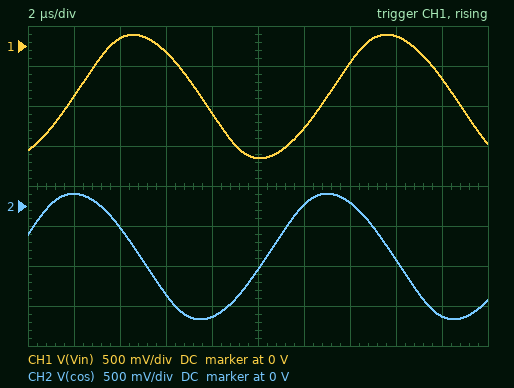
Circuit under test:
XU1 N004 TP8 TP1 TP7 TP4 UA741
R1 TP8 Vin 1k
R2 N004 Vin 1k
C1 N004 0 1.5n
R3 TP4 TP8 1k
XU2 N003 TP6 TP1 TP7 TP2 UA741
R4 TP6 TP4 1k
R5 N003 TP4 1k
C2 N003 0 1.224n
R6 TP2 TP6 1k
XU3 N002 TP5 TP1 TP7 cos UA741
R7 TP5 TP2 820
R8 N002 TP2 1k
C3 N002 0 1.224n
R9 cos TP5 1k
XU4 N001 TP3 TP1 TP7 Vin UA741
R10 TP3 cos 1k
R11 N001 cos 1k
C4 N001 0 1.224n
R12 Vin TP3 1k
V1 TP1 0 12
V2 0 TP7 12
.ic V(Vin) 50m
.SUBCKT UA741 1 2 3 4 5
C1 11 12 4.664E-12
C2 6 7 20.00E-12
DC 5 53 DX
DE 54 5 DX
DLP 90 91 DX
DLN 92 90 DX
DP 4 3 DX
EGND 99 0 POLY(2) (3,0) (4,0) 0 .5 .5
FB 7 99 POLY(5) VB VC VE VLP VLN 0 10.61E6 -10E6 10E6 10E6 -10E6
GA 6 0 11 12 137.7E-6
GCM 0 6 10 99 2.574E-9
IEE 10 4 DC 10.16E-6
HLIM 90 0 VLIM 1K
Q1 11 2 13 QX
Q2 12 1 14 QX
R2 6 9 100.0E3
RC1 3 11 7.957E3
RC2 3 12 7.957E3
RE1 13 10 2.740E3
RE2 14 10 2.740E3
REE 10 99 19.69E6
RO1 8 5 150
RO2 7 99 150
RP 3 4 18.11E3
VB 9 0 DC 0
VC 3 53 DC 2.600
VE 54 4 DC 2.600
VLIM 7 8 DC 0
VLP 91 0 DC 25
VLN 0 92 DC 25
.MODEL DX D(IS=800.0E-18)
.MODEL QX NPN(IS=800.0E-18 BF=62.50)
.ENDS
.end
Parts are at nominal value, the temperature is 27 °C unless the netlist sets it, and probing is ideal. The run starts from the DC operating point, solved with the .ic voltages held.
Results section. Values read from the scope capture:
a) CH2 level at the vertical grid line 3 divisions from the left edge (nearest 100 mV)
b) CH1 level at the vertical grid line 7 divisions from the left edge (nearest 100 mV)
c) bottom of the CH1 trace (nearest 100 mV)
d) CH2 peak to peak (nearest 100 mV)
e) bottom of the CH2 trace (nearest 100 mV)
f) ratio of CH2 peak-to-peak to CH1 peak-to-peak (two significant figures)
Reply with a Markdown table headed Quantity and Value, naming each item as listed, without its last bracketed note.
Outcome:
| Quantity | Value |
|---|---|
| CH2 level at the vertical grid line 3 divisions from the left edge | -1.1 V |
| CH1 level at the vertical grid line 7 divisions from the left edge | -200 mV |
| bottom of the CH1 trace | -1.4 V |
| CH2 peak to peak | 1.6 V |
| bottom of the CH2 trace | -1.4 V |
| ratio of CH2 peak-to-peak to CH1 peak-to-peak | 1.0 |
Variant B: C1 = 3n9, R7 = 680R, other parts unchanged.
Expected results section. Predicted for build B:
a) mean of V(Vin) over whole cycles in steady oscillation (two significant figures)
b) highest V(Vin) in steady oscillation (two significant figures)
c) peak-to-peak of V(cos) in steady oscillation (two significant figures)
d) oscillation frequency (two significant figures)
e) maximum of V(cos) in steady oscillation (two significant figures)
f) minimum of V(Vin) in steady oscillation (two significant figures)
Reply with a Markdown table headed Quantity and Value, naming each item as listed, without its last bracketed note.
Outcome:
| Quantity | Value |
|---|---|
| mean of V(Vin) over whole cycles in steady oscillation | -390 mV |
| highest V(Vin) in steady oscillation | 720 mV |
| peak-to-peak of V(cos) in steady oscillation | 2.3 V |
| oscillation frequency | 70 kHz |
| maximum of V(cos) in steady oscillation | 760 mV |
| minimum of V(Vin) in steady oscillation | -1.5 V |
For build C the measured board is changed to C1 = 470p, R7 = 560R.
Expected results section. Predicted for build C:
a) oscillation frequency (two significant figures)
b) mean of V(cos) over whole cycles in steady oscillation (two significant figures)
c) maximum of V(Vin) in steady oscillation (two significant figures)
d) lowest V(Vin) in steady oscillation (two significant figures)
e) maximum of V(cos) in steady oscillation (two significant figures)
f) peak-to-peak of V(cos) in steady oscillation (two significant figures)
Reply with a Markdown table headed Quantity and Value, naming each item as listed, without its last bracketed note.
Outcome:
| Quantity | Value |
|---|---|
| oscillation frequency | 98 kHz |
| mean of V(cos) over whole cycles in steady oscillation | -600 mV |
| maximum of V(Vin) in steady oscillation | 200 mV |
| lowest V(Vin) in steady oscillation | -1.4 V |
| maximum of V(cos) in steady oscillation | 250 mV |
| peak-to-peak of V(cos) in steady oscillation | 1.7 V |
